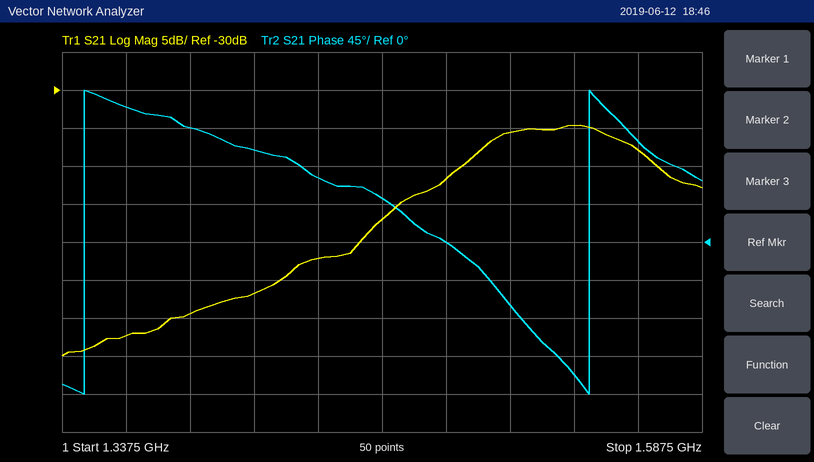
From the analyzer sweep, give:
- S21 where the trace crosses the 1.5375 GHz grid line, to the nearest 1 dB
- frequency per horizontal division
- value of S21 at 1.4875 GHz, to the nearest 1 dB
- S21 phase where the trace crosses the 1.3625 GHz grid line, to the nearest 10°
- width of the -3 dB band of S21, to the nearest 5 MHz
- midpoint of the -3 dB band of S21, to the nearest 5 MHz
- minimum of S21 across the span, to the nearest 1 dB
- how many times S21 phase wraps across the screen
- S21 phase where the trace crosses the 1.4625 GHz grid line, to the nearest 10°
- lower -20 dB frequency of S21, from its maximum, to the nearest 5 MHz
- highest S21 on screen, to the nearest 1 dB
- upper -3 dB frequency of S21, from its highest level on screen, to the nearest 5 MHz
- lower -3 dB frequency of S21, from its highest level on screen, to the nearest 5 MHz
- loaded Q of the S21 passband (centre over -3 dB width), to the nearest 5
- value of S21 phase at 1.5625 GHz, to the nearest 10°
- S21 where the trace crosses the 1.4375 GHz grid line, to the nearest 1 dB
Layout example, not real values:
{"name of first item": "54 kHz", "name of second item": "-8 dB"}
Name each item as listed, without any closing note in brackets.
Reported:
{"S21 where the trace crosses the 1.5375 GHz grid line, to the nearest 1 dB": "-35 dB", "frequency per horizontal division": "25 MHz", "value of S21 at 1.4875 GHz, to the nearest 1 dB": "-42 dB", "S21 phase where the trace crosses the 1.3625 GHz grid line, to the nearest 10°": "160°", "width of the -3 dB band of S21, to the nearest 5 MHz": "60 MHz", "midpoint of the -3 dB band of S21, to the nearest 5 MHz": "1.530 GHz", "minimum of S21 across the span, to the nearest 1 dB": "-65 dB", "how many times S21 phase wraps across the screen": "2", "S21 phase where the trace crosses the 1.4625 GHz grid line, to the nearest 10°": "50°", "lower -20 dB frequency of S21, from its maximum, to the nearest 5 MHz": "1.425 GHz", "highest S21 on screen, to the nearest 1 dB": "-35 dB", "upper -3 dB frequency of S21, from its highest level on screen, to the nearest 5 MHz": "1.560 GHz", "lower -3 dB frequency of S21, from its highest level on screen, to the nearest 5 MHz": "1.500 GHz", "loaded Q of the S21 passband (centre over -3 dB width), to the nearest 5": "25", "value of S21 phase at 1.5625 GHz, to the nearest 10°": "120°", "S21 where the trace crosses the 1.4375 GHz grid line, to the nearest 1 dB": "-52 dB"}
